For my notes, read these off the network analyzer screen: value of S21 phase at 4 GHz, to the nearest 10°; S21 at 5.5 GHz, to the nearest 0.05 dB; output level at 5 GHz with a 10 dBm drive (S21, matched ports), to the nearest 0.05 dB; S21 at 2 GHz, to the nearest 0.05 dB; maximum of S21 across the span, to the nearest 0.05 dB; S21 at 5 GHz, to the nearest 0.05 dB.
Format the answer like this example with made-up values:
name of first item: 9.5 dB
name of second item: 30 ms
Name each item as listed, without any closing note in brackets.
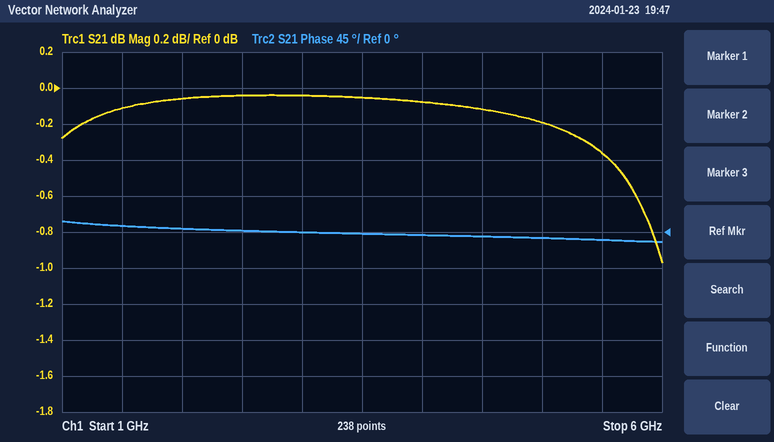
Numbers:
value of S21 phase at 4 GHz, to the nearest 10°: 0°
S21 at 5.5 GHz, to the nearest 0.05 dB: -0.35 dB
output level at 5 GHz with a 10 dBm drive (S21, matched ports), to the nearest 0.05 dB: 9.80 dBm
S21 at 2 GHz, to the nearest 0.05 dB: -0.05 dB
maximum of S21 across the span, to the nearest 0.05 dB: -0.05 dB
S21 at 5 GHz, to the nearest 0.05 dB: -0.20 dB
